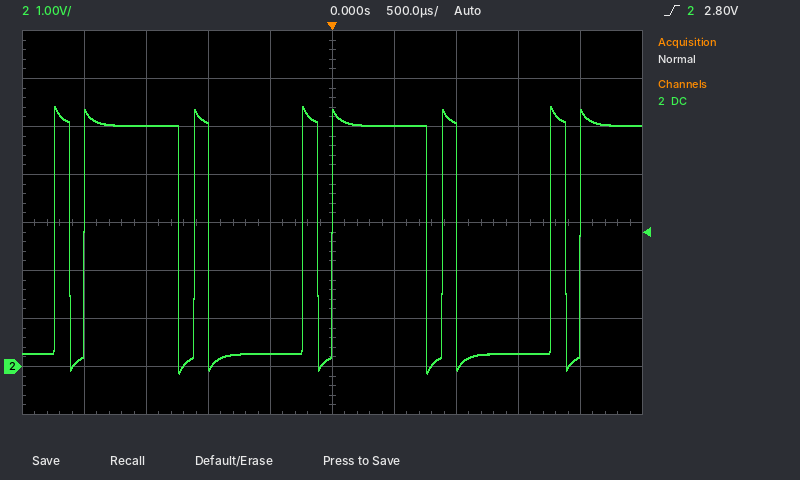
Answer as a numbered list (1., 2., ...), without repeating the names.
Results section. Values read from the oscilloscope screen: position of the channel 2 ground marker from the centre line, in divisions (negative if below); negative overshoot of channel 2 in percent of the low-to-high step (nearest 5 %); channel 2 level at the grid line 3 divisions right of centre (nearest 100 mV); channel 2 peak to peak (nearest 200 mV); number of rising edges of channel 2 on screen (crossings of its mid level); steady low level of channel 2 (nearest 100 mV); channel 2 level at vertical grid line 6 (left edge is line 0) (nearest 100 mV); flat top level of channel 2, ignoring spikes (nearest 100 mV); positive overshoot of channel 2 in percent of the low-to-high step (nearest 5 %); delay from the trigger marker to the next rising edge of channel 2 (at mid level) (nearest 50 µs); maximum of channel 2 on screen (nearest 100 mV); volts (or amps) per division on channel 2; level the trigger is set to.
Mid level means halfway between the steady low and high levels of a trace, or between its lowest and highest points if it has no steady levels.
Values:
1. -3.0 div
2. 10 %
3. 300 mV
4. 5.6 V
5. 8
6. 300 mV
7. 5.0 V
8. 5.0 V
9. 10 %
10. 900 µs
11. 5.4 V
12. 1 V
13. 2.80 V
